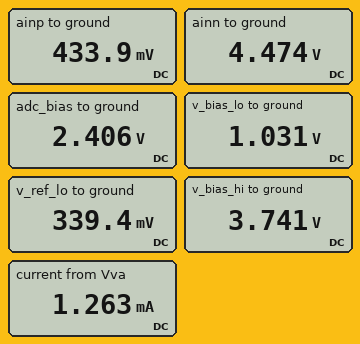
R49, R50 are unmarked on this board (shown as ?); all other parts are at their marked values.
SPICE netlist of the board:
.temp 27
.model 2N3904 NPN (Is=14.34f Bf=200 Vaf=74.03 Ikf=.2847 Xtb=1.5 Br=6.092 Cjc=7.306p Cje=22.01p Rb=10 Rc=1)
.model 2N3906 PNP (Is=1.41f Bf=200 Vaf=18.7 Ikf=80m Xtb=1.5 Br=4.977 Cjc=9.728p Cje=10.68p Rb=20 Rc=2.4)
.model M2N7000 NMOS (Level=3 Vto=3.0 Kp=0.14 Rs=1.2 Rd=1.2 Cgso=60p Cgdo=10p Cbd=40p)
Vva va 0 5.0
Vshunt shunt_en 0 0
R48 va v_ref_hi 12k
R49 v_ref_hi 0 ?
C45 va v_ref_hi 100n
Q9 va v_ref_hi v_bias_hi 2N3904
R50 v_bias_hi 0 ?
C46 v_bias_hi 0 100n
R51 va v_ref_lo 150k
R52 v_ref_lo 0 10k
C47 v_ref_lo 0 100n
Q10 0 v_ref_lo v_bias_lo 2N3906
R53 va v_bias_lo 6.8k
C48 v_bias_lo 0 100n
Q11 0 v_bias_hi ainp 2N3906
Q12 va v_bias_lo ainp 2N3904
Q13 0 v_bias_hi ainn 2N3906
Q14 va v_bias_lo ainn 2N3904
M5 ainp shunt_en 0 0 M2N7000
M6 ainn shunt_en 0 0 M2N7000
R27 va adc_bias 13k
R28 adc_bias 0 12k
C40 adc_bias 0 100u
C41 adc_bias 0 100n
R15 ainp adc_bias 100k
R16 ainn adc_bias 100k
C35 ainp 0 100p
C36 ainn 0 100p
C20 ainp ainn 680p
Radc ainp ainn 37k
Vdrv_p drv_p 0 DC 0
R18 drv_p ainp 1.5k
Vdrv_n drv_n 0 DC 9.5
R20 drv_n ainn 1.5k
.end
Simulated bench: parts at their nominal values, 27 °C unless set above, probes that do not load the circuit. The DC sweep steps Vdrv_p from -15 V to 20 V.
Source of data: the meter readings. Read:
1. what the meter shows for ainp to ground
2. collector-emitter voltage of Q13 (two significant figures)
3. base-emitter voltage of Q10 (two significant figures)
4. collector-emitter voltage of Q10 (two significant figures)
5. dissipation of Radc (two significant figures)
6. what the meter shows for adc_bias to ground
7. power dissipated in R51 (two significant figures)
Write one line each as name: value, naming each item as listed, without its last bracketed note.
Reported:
what the meter shows for ainp to ground: 433.9 mV
collector-emitter voltage of Q13: -4.5 V
base-emitter voltage of Q10: -690 mV
collector-emitter voltage of Q10: -1.0 V
dissipation of Radc: 440 µW
what the meter shows for adc_bias to ground: 2.406 V
power dissipated in R51: 140 µW
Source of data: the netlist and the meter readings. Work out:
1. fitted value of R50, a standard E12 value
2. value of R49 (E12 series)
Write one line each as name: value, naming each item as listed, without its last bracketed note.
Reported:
fitted value of R50, a standard E12 value: 15 kΩ
value of R49: 82 kΩ
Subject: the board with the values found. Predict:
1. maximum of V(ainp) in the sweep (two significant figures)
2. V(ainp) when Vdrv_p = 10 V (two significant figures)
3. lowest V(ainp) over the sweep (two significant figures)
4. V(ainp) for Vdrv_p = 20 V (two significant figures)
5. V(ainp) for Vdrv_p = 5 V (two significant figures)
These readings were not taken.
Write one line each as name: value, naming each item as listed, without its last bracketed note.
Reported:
maximum of V(ainp) in the sweep: 4.5 V
V(ainp) when Vdrv_p = 10 V: 4.5 V
lowest V(ainp) over the sweep: 320 mV
V(ainp) for Vdrv_p = 20 V: 4.5 V
V(ainp) for Vdrv_p = 5 V: 4.4 V
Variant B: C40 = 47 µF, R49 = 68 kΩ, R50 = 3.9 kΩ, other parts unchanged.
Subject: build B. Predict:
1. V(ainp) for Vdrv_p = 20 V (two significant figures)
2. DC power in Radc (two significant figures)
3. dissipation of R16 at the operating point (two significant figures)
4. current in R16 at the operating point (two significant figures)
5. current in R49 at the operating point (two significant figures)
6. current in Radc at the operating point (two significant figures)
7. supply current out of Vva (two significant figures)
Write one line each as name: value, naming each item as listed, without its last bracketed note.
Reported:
V(ainp) for Vdrv_p = 20 V: 4.3 V
DC power in Radc: 400 µW
dissipation of R16 at the operating point: 36 µW
current in R16 at the operating point: 19 µA
current in R49 at the operating point: 62 µA
current in Radc at the operating point: 100 µA
supply current out of Vva: 1.9 mA
